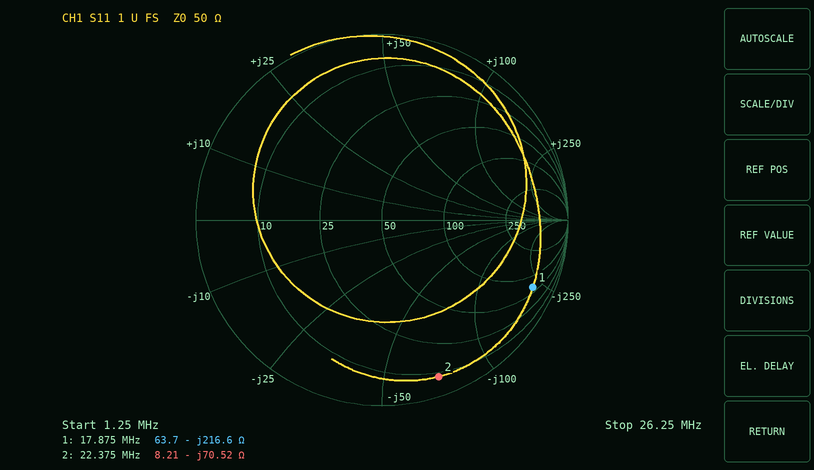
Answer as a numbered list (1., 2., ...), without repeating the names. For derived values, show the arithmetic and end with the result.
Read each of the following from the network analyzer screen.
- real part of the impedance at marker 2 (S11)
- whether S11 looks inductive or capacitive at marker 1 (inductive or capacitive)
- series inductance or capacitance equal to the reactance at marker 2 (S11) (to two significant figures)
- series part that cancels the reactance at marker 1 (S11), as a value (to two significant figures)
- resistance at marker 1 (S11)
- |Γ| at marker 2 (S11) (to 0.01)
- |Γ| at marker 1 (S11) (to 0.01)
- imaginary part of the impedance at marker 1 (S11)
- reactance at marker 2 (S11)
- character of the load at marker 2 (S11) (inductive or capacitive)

1. 8.21 Ω
2. capacitive
3. C = 1/(2π × 22.375 MHz × 70.52 Ω) ≈ 101 pF, so 100 pF to two significant figures
4. L = 216.6 Ω/(2π × 17.875 MHz) ≈ 1.9 µH
5. 63.7 Ω
6. 0.90
7. 0.89
8. -216.6 Ω
9. -70.52 Ω
10. capacitive
